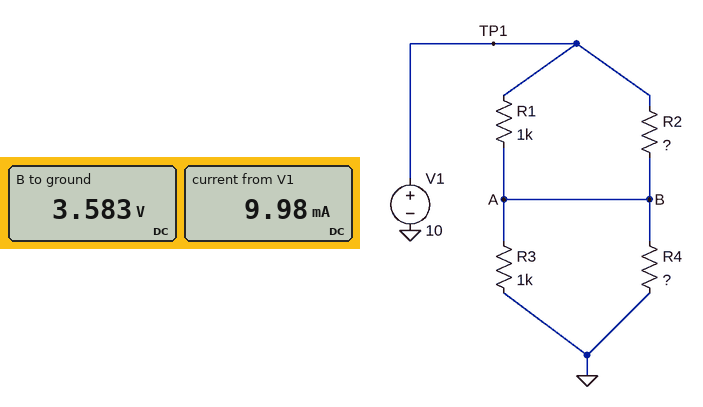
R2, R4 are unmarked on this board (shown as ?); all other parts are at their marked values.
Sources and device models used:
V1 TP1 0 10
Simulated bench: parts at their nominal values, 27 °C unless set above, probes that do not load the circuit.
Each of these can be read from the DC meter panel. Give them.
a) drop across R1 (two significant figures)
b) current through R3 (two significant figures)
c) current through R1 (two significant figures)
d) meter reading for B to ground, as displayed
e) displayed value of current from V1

6.4 V
3.6 mA
6.4 mA
3.583 V
9.98 mA
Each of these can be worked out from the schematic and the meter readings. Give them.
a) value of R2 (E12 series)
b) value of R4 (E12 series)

1.8 kΩ
560 Ω
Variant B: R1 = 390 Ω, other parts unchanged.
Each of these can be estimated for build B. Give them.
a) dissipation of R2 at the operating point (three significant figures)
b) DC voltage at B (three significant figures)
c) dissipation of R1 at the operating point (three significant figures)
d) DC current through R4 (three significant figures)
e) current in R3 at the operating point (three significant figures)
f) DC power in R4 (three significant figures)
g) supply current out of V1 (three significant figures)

12.4 mW
5.28 V
57.1 mW
9.43 mA
5.28 mA
49.8 mW
14.7 mA
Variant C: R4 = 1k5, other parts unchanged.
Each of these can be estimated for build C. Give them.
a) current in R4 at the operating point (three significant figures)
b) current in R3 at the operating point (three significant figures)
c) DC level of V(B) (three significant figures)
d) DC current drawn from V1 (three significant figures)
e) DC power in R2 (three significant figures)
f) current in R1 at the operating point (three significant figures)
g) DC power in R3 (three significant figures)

3.22 mA
4.83 mA
4.83 V
8.05 mA
14.9 mW
5.17 mA
23.3 mW
